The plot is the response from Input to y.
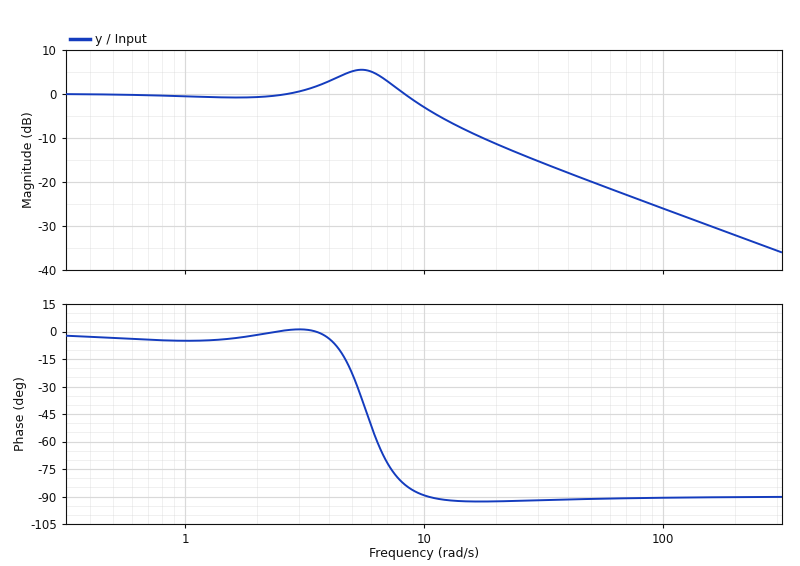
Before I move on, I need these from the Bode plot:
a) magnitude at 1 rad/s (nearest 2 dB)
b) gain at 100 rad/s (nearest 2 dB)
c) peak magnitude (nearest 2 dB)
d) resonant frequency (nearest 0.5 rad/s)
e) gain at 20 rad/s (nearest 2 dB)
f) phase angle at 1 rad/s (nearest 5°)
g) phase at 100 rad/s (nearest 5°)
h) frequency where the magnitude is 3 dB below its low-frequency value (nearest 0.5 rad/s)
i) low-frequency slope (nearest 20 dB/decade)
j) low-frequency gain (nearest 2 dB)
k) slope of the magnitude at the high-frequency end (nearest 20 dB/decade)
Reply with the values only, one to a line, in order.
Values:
0 dB
-26 dB
6 dB
5.5 rad/s
-12 dB
-5°
-90°
10.0 rad/s
0 dB/decade
0 dB
-20 dB/decade
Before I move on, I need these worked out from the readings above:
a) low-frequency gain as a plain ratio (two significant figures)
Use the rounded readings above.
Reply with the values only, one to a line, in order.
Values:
1.0
